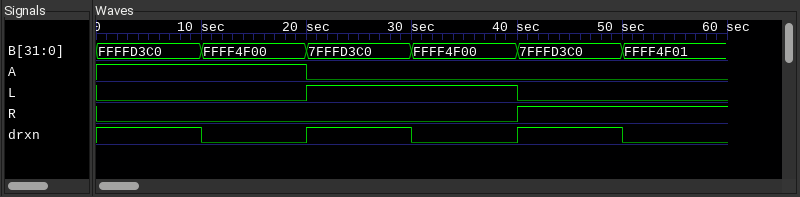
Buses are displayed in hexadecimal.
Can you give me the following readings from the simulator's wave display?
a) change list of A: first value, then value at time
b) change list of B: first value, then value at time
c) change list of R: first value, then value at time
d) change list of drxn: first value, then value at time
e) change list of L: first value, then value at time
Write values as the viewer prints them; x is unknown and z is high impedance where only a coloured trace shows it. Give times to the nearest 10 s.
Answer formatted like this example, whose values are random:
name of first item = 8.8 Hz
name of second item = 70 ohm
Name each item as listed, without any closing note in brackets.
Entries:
change list of A: first value, then value at time = 1, 0 at 20 s
change list of B: first value, then value at time = FFFFD3C0, FFFF4F00 at 10 s, 7FFFD3C0 at 20 s, FFFF4F00 at 30 s, 7FFFD3C0 at 40 s, FFFF4F01 at 50 s
change list of R: first value, then value at time = 0, 1 at 40 s
change list of drxn: first value, then value at time = 1, 0 at 10 s, 1 at 20 s, 0 at 30 s, 1 at 40 s, 0 at 50 s
change list of L: first value, then value at time = 0, 1 at 20 s, 0 at 40 s
